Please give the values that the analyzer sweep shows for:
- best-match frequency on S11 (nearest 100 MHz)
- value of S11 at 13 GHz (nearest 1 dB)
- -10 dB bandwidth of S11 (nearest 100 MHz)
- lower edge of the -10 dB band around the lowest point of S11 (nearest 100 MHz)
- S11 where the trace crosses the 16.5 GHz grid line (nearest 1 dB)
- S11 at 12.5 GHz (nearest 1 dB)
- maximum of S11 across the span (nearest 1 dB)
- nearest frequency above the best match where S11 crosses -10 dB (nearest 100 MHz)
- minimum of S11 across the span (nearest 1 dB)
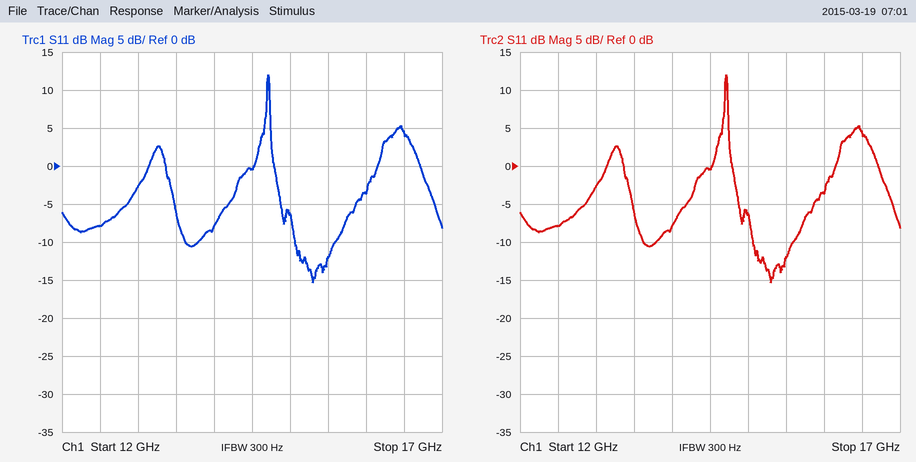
15.3 GHz
-3 dB
500 MHz
15.1 GHz
4 dB
-8 dB
12 dB
15.6 GHz
-15 dB
